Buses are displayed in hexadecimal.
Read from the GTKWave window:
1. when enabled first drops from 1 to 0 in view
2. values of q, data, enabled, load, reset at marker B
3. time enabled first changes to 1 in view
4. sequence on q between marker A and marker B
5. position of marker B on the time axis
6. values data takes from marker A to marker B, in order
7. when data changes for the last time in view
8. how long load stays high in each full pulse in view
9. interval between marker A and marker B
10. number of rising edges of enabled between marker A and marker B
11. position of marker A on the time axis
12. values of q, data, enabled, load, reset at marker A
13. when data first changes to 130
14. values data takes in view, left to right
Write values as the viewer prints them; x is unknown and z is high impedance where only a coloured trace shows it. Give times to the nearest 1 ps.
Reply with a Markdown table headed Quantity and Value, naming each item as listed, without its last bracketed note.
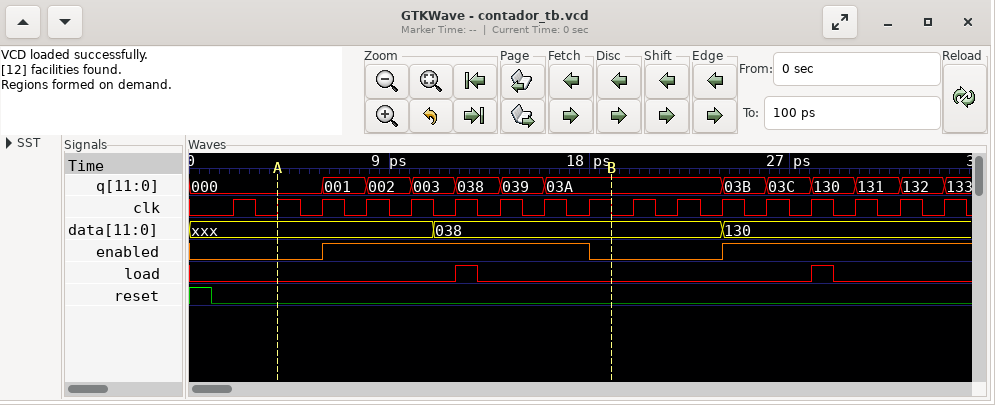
| Quantity | Value |
|---|---|
| when enabled first drops from 1 to 0 in view | 18 ps |
| values of q, data, enabled, load, reset at marker B | q=03A, data=038, enabled=0, load=0, reset=0 |
| time enabled first changes to 1 in view | 6 ps |
| sequence on q between marker A and marker B | 000, 001, 002, 003, 038, 039, 03A |
| position of marker B on the time axis | 19 ps |
| values data takes from marker A to marker B, in order | xxx, 038 |
| when data changes for the last time in view | 24 ps |
| how long load stays high in each full pulse in view | 1 ps, 1 ps |
| interval between marker A and marker B | 15 ps |
| number of rising edges of enabled between marker A and marker B | 1 |
| position of marker A on the time axis | 4 ps |
| values of q, data, enabled, load, reset at marker A | q=000, data=xxx, enabled=0, load=0, reset=0 |
| when data first changes to 130 | 24 ps |
| values data takes in view, left to right | xxx, 038, 130 |
